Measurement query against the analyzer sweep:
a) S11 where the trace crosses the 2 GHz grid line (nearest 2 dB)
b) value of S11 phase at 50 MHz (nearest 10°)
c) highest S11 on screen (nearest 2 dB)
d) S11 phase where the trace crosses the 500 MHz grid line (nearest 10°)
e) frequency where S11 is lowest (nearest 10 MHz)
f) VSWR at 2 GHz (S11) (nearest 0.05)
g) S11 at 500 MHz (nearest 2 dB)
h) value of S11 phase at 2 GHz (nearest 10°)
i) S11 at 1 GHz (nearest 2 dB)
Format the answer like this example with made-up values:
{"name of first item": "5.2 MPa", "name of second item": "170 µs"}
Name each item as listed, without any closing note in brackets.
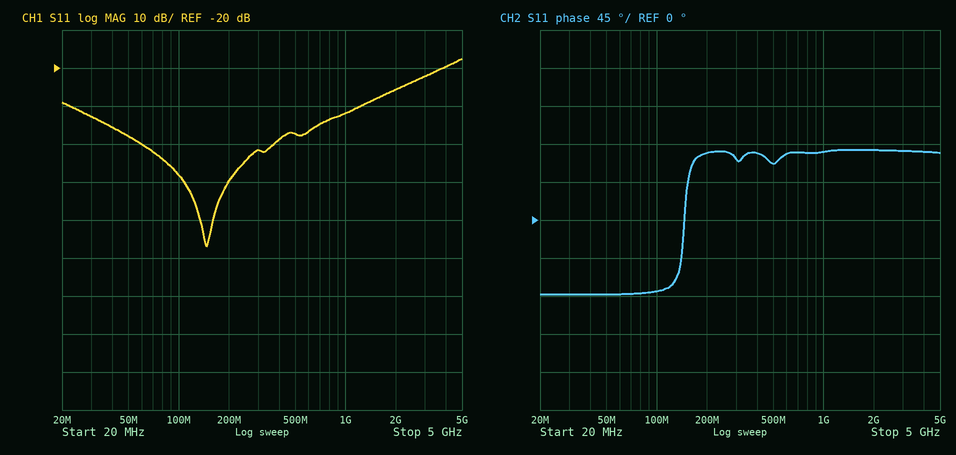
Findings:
{"S11 where the trace crosses the 2 GHz grid line": "-26 dB", "value of S11 phase at 50 MHz": "-90°", "highest S11 on screen": "-18 dB", "S11 phase where the trace crosses the 500 MHz grid line": "70°", "frequency where S11 is lowest": "150 MHz", "VSWR at 2 GHz (S11)": "1.10", "S11 at 500 MHz": "-38 dB", "value of S11 phase at 2 GHz": "80°", "S11 at 1 GHz": "-32 dB"}
